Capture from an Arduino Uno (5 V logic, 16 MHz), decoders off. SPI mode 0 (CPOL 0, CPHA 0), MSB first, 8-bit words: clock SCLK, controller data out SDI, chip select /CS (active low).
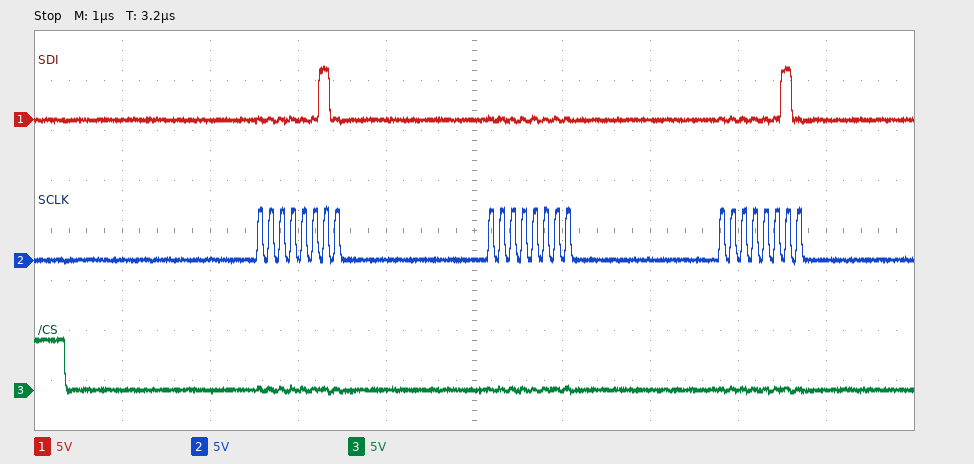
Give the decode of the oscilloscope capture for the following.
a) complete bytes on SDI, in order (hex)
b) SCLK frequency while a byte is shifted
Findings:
02 00 02
8 MHz
